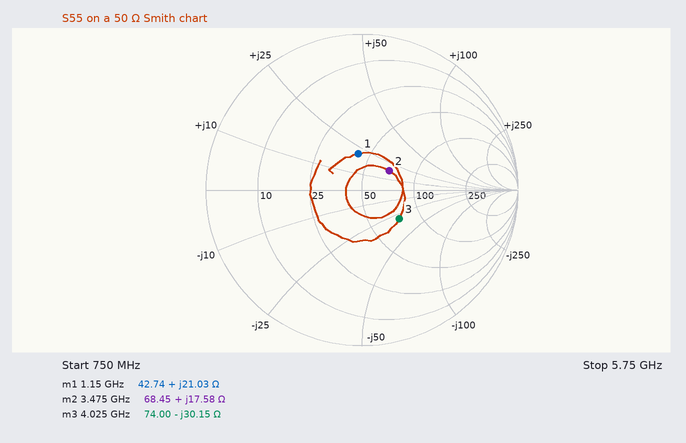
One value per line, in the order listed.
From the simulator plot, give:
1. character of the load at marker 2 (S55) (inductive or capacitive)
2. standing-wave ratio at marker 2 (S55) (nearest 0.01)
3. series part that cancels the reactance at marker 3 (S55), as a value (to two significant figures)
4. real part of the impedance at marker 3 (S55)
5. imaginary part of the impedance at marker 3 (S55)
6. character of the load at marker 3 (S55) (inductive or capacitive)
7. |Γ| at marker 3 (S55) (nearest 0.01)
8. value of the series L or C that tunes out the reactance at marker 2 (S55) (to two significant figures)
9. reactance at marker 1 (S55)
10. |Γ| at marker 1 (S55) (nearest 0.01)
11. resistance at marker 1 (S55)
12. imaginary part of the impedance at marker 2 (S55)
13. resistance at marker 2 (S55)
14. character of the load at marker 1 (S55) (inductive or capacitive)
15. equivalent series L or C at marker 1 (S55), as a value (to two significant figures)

inductive
1.54
1.2 nH
74.00 Ω
-30.15 Ω
capacitive
0.30
2.6 pF
+21.03 Ω
0.23
42.74 Ω
+17.58 Ω
68.45 Ω
inductive
2.9 nH
